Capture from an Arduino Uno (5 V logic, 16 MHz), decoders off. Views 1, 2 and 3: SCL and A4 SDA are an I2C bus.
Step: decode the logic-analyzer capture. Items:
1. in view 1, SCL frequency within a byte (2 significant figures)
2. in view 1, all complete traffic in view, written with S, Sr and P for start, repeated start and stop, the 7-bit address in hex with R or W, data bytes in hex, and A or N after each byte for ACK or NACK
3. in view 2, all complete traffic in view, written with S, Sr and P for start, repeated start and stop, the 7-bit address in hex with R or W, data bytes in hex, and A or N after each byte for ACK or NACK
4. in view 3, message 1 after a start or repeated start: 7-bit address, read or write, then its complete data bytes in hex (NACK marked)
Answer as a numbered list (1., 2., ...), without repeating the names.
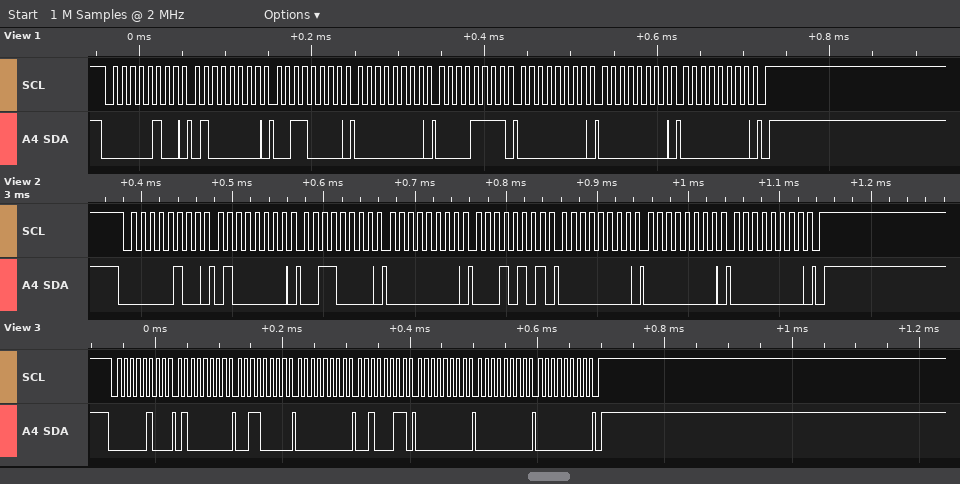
1. 100 kHz
2. S 02W A 40 A 30 A 00 A 0F A 00 A 00 A 00 A P
3. S 02W A 40 A 30 A 00 A 15 A 00 A 00 A 00 A P
4. 0x02 write: 40 30 00 23 00 00 00
